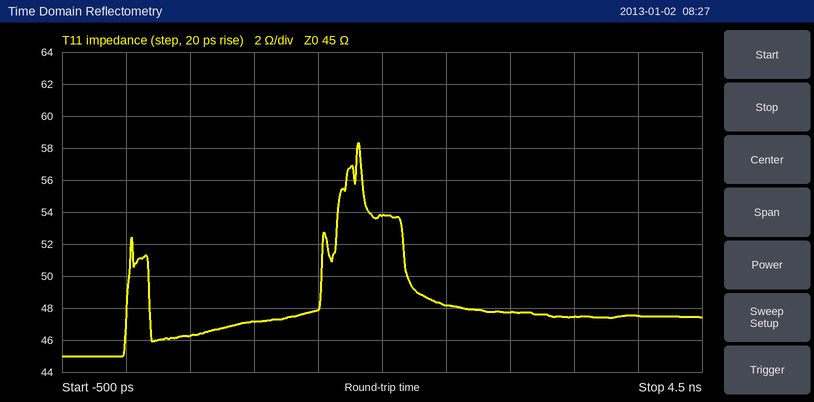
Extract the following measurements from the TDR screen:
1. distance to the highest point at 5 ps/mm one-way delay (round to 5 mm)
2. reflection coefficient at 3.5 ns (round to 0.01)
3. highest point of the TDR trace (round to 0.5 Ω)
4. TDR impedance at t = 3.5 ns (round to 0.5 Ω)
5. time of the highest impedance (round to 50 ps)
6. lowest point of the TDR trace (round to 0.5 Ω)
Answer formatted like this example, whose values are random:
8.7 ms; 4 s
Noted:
180 mm; +0.03; 58.5 Ω; 47.5 Ω; 1.80 ns; 45.0 Ω
